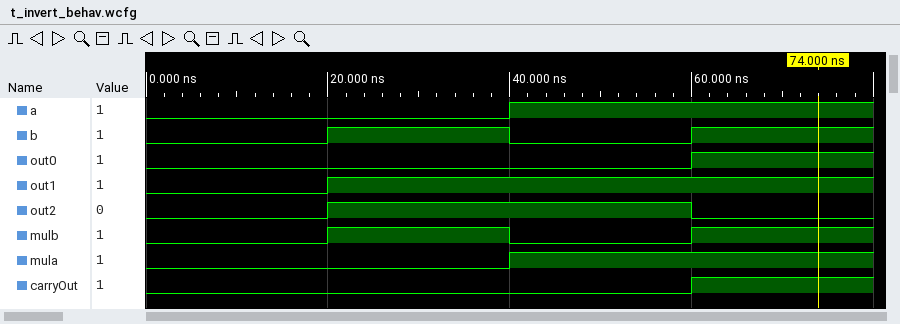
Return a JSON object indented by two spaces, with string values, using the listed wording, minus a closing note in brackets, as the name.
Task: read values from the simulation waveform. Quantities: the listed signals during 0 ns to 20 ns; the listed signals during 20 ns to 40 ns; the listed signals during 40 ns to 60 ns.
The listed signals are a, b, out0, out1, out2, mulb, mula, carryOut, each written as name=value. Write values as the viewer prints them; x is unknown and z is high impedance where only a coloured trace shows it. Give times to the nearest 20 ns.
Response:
{
  "the listed signals during 0 ns to 20 ns": "a=0, b=0, out0=0, out1=0, out2=0, mulb=0, mula=0, carryOut=0",
  "the listed signals during 20 ns to 40 ns": "a=0, b=1, out0=0, out1=1, out2=1, mulb=1, mula=0, carryOut=0",
  "the listed signals during 40 ns to 60 ns": "a=1, b=0, out0=0, out1=1, out2=1, mulb=0, mula=1, carryOut=0"
}
